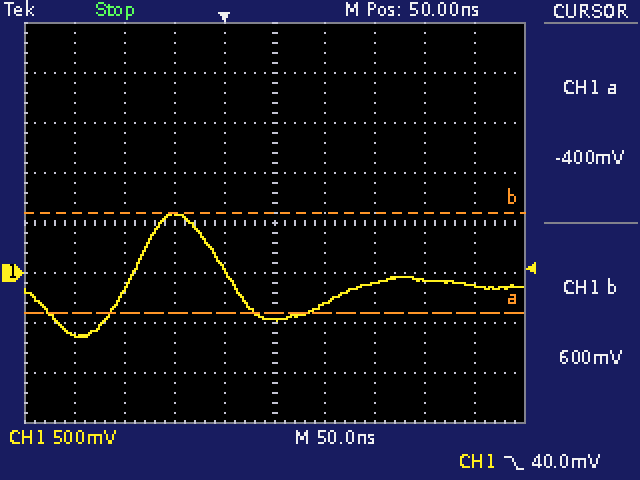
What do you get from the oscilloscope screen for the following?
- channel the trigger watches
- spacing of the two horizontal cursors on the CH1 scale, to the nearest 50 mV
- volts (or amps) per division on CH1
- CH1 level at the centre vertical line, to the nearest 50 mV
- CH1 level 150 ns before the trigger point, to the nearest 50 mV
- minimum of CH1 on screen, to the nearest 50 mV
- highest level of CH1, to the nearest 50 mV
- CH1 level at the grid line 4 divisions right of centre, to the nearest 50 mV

CH1
1.00 V
500 mV
-450 mV
-600 mV
-650 mV
600 mV
-150 mV
